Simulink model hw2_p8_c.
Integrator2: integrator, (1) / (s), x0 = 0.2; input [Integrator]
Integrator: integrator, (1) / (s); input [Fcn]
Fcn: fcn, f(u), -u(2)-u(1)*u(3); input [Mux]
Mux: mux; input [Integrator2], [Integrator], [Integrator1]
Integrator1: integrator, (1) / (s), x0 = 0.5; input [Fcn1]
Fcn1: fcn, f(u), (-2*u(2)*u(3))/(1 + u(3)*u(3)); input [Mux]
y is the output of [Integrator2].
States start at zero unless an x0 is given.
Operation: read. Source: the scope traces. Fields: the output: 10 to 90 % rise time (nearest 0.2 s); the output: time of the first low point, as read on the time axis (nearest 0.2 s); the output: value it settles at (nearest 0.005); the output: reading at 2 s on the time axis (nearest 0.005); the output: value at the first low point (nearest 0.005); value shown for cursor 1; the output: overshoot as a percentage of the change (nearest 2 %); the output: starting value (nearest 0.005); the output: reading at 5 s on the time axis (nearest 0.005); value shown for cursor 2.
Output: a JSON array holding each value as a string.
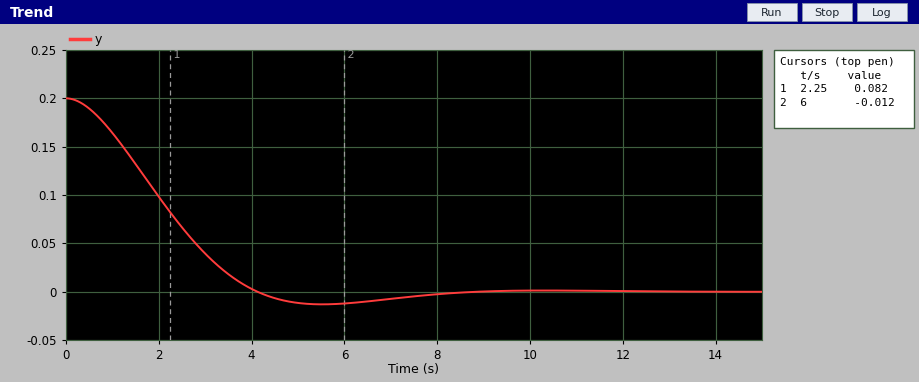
["2.8 s", "5.6 s", "0.000", "0.100", "-0.015", "0.082", "6 %", "0.200", "-0.010", "-0.012"]
